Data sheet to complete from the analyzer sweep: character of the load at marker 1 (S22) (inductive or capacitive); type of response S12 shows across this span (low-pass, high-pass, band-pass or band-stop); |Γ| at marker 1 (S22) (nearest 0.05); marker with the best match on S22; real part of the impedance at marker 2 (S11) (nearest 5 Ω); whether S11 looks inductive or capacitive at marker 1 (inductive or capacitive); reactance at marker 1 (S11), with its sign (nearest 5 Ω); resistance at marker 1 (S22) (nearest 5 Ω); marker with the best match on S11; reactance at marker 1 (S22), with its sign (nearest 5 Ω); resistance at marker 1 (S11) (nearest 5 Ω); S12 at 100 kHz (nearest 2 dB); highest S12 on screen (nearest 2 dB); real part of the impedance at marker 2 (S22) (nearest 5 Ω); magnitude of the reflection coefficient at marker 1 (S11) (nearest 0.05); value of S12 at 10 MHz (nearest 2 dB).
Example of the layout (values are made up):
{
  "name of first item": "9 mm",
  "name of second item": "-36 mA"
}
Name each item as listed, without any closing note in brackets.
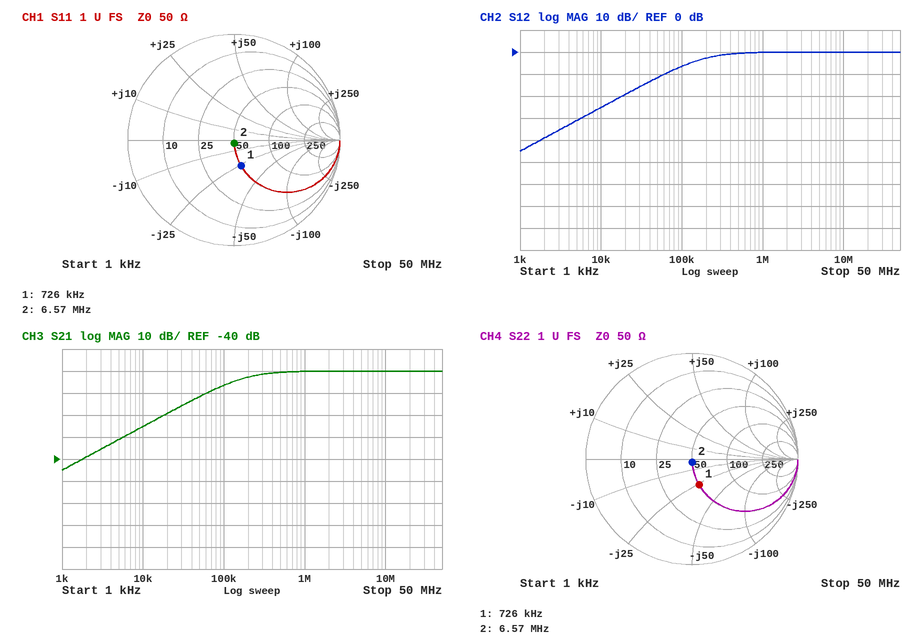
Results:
{
  "character of the load at marker 1 (S22)": "capacitive",
  "type of response S12 shows across this span": "high-pass",
  "|Γ| at marker 1 (S22)": "0.25",
  "marker with the best match on S22": "marker 2",
  "real part of the impedance at marker 2 (S11)": "50 Ω",
  "whether S11 looks inductive or capacitive at marker 1": "capacitive",
  "reactance at marker 1 (S11), with its sign": "-25 Ω",
  "resistance at marker 1 (S22)": "50 Ω",
  "marker with the best match on S11": "marker 2",
  "reactance at marker 1 (S22), with its sign": "-25 Ω",
  "resistance at marker 1 (S11)": "50 Ω",
  "S12 at 100 kHz": "-6 dB",
  "highest S12 on screen": "0 dB",
  "real part of the impedance at marker 2 (S22)": "50 Ω",
  "magnitude of the reflection coefficient at marker 1 (S11)": "0.25",
  "value of S12 at 10 MHz": "0 dB"
}
